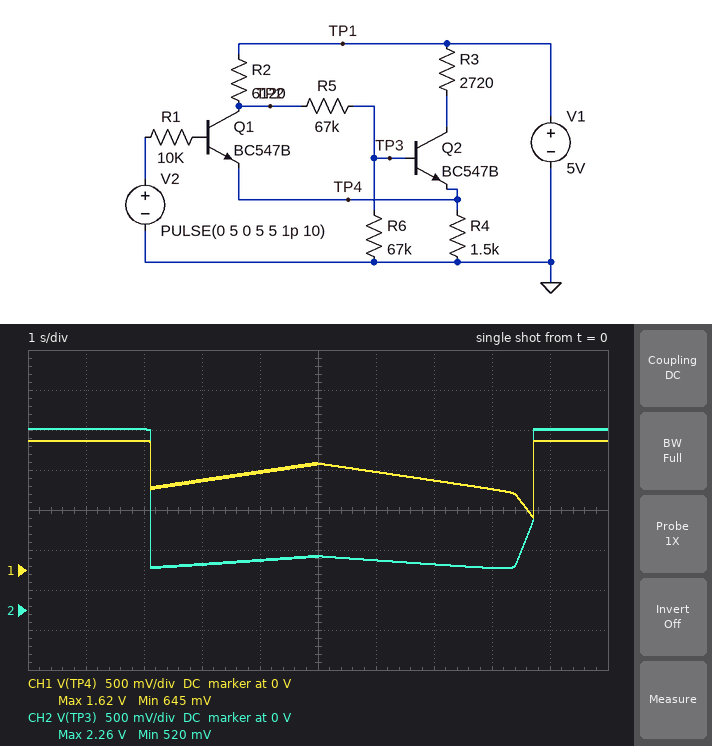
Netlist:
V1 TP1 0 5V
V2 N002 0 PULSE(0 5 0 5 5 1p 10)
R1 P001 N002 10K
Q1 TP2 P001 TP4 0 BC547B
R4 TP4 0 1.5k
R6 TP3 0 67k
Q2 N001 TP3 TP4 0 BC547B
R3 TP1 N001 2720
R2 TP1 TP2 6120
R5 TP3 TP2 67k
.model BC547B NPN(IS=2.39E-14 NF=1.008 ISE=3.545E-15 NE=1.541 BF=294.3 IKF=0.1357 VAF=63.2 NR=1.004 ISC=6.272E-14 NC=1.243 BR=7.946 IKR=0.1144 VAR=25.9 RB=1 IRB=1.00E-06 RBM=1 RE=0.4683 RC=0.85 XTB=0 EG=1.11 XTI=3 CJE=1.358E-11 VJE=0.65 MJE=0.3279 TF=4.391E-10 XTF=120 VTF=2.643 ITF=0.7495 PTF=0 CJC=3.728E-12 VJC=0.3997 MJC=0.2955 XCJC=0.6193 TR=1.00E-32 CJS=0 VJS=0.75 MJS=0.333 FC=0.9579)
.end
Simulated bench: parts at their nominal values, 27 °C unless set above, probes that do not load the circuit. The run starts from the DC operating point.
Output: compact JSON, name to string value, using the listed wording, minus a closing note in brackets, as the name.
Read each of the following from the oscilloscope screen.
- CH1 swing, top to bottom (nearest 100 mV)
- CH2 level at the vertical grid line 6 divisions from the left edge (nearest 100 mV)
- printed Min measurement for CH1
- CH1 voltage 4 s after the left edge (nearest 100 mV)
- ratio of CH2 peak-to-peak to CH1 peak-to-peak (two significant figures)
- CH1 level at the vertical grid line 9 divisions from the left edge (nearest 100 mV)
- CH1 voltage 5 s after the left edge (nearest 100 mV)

{"CH1 swing, top to bottom": "1.0 V", "CH2 level at the vertical grid line 6 divisions from the left edge": "600 mV", "printed Min measurement for CH1": "645 mV", "CH1 voltage 4 s after the left edge": "1.2 V", "ratio of CH2 peak-to-peak to CH1 peak-to-peak": "1.8", "CH1 level at the vertical grid line 9 divisions from the left edge": "1.6 V", "CH1 voltage 5 s after the left edge": "1.3 V"}
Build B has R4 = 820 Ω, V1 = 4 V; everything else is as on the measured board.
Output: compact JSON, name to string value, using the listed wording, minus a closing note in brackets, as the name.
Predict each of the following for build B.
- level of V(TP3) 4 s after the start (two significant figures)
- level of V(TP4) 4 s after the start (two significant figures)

{"level of V(TP3) 4 s after the start": "340 mV", "level of V(TP4) 4 s after the start": "660 mV"}
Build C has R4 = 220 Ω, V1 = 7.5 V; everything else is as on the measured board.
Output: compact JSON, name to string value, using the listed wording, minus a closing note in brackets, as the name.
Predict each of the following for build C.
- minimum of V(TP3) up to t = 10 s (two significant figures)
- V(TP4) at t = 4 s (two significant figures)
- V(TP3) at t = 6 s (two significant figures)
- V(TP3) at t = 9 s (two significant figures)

{"minimum of V(TP3) up to t = 10 s": "160 mV", "V(TP4) at t = 4 s": "320 mV", "V(TP3) at t = 6 s": "170 mV", "V(TP3) at t = 9 s": "180 mV"}
